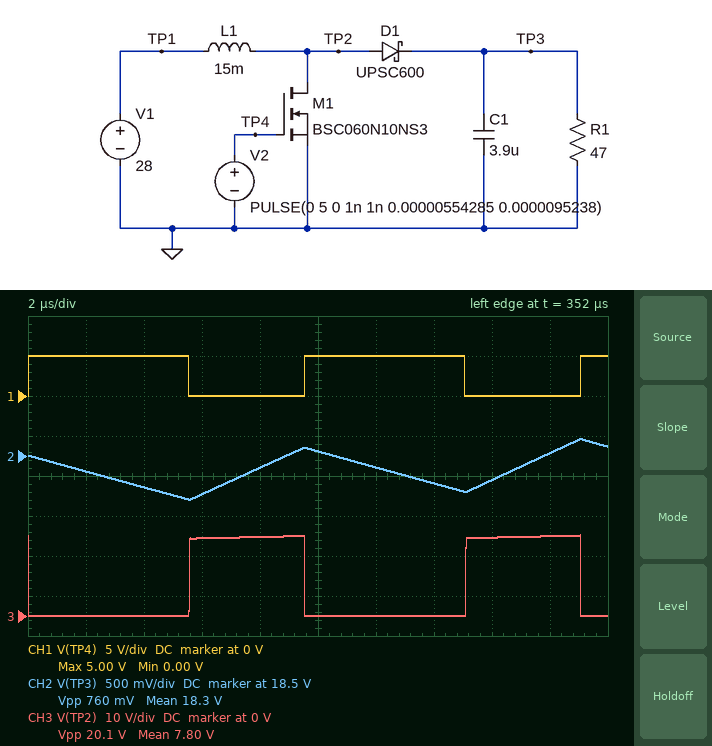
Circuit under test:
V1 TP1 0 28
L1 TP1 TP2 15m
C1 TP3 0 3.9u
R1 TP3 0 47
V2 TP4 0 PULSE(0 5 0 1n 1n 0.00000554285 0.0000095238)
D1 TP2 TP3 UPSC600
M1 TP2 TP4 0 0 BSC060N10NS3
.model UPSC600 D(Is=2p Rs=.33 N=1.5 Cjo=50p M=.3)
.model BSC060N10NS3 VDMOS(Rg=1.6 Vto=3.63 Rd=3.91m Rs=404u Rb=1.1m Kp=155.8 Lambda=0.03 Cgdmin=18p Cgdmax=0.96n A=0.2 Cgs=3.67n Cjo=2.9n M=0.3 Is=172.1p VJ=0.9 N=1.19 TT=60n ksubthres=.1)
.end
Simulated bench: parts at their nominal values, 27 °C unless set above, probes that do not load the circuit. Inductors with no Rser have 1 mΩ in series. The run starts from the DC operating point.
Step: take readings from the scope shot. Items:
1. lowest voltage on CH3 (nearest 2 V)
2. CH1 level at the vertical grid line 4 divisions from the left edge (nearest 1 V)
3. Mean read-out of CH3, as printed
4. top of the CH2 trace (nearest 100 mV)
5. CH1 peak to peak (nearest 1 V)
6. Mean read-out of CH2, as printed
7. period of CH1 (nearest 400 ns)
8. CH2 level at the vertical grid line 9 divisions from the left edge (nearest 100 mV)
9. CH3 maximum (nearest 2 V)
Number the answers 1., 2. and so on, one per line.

1. 0 V
2. 0 V
3. 7.80 V
4. 18.7 V
5. 5 V
6. 18.3 V
7. 9.6 µs
8. 18.5 V
9. 20 V
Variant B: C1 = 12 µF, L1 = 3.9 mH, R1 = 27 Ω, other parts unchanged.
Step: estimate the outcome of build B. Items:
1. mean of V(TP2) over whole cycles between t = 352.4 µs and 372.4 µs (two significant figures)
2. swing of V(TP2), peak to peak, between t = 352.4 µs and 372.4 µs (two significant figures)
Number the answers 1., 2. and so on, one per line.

1. 11 V
2. 26 V
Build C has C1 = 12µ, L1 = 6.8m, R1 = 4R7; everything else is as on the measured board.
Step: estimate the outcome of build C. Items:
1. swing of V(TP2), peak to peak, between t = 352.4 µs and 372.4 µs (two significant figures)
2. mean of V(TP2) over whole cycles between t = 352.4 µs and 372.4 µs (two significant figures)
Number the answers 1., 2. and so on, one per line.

1. 16 V
2. 6.6 V
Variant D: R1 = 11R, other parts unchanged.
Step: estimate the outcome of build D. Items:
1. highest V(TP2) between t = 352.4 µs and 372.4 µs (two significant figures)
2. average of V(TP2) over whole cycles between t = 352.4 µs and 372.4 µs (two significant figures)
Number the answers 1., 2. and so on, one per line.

1. 16 V
2. 6.3 V
